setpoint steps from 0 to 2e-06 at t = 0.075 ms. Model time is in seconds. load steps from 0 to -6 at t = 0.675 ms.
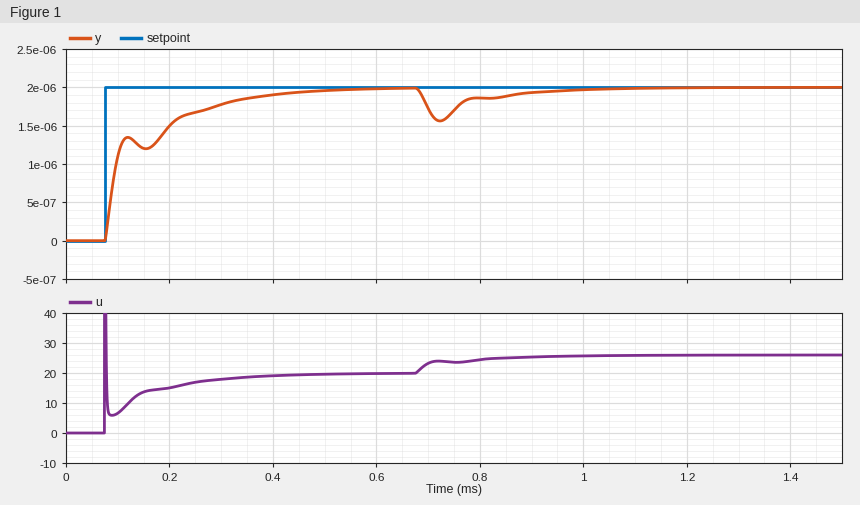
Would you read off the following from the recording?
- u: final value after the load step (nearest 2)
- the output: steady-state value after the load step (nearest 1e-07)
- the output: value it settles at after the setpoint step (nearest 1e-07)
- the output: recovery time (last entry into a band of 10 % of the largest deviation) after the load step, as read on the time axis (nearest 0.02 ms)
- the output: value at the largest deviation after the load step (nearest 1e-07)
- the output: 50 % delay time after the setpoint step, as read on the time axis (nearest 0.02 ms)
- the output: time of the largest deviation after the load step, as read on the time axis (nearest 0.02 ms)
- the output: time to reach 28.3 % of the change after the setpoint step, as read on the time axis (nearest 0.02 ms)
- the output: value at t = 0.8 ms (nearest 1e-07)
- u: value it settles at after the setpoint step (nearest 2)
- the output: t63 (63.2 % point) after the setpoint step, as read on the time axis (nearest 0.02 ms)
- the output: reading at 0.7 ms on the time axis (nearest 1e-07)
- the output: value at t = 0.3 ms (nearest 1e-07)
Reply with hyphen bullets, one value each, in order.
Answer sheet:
- 26
- 0.0000020
- 0.0000020
- 0.96 ms
- 0.0000016
- 0.10 ms
- 0.72 ms
- 0.08 ms
- 0.0000019
- 20
- 0.10 ms
- 0.0000017
- 0.0000018
